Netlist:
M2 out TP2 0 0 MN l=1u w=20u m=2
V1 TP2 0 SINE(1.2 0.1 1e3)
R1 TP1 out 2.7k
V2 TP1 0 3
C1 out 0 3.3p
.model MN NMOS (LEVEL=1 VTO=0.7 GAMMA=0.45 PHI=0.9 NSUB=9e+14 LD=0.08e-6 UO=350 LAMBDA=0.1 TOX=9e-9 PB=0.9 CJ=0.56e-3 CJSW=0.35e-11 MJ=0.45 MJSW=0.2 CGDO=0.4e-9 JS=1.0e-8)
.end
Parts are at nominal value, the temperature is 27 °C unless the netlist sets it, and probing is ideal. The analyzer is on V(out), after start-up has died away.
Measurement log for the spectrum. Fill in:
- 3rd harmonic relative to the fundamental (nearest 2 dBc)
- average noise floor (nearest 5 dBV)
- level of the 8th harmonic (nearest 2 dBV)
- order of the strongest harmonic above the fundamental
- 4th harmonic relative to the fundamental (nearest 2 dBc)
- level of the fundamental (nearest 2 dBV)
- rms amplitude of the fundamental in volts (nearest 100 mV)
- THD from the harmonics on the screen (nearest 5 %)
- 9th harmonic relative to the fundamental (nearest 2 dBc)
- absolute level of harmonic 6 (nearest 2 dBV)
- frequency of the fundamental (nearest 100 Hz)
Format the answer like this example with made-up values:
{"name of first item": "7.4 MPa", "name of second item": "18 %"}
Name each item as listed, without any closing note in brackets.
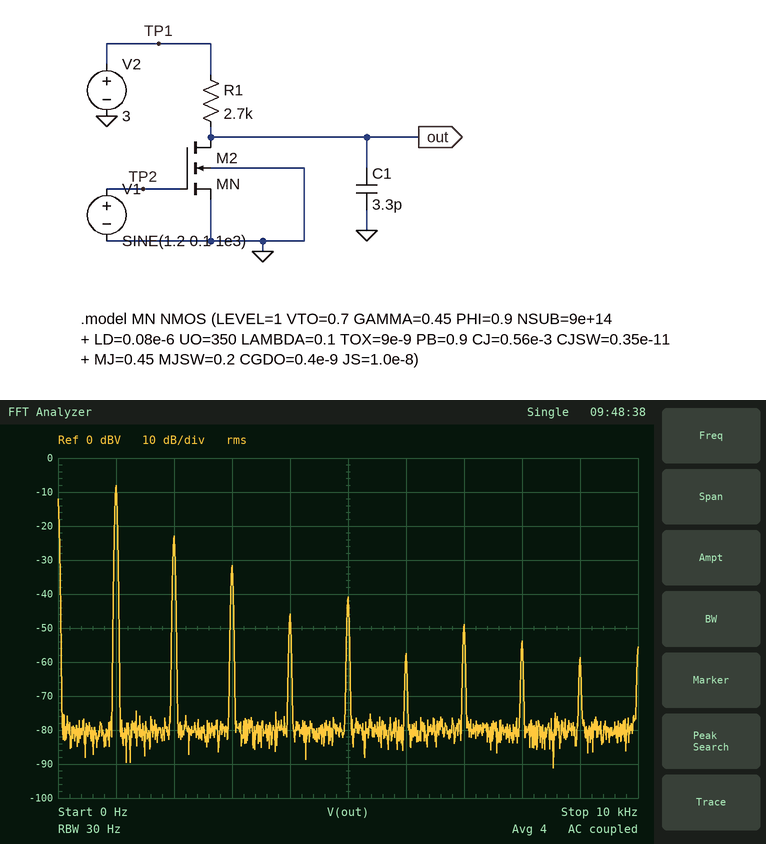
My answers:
{"3rd harmonic relative to the fundamental": "-24 dBc", "average noise floor": "-80 dBV", "level of the 8th harmonic": "-54 dBV", "order of the strongest harmonic above the fundamental": "2", "4th harmonic relative to the fundamental": "-38 dBc", "level of the fundamental": "-8 dBV", "rms amplitude of the fundamental in volts": "400 mV", "THD from the harmonics on the screen": "20 %", "9th harmonic relative to the fundamental": "-50 dBc", "absolute level of harmonic 6": "-58 dBV", "frequency of the fundamental": "1.0 kHz"}
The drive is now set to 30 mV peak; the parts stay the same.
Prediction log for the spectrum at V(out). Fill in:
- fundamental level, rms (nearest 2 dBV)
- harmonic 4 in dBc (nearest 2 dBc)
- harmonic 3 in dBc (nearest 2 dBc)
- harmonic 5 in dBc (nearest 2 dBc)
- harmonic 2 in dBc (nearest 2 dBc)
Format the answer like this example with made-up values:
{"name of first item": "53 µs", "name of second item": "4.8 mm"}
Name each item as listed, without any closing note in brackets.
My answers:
{"fundamental level, rms": "-16 dBV", "harmonic 4 in dBc": "-40 dBc", "harmonic 3 in dBc": "-36 dBc", "harmonic 5 in dBc": "-44 dBc", "harmonic 2 in dBc": "-38 dBc"}
